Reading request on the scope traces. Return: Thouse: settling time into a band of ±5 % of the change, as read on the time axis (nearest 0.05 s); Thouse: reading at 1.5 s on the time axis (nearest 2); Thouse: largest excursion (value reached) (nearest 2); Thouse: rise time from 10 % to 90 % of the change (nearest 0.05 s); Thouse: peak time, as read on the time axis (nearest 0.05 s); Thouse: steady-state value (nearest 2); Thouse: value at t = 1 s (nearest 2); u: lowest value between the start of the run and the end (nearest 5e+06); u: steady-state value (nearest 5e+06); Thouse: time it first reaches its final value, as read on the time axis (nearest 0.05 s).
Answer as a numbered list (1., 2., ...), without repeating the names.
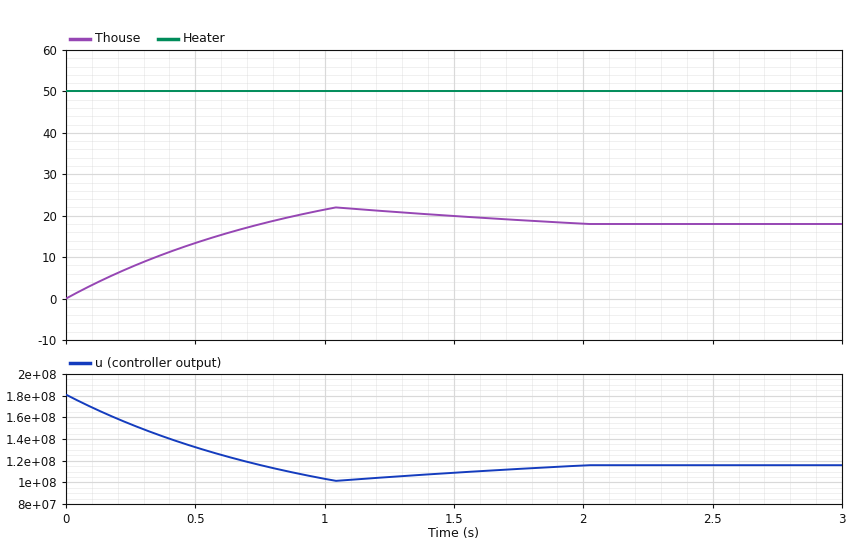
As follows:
1. 1.75 s
2. 20
3. 22
4. 0.60 s
5. 1.05 s
6. 18
7. 22
8. 100000000
9. 115000000
10. 0.75 s
